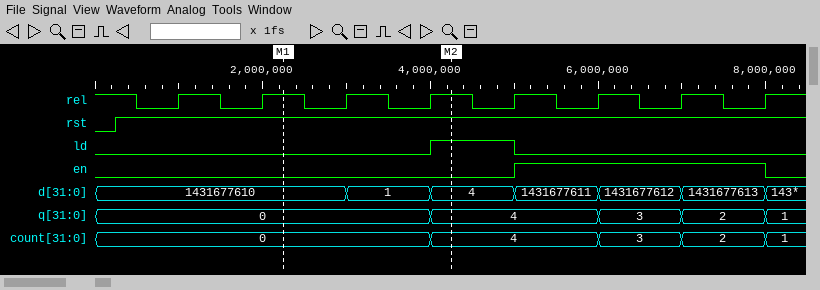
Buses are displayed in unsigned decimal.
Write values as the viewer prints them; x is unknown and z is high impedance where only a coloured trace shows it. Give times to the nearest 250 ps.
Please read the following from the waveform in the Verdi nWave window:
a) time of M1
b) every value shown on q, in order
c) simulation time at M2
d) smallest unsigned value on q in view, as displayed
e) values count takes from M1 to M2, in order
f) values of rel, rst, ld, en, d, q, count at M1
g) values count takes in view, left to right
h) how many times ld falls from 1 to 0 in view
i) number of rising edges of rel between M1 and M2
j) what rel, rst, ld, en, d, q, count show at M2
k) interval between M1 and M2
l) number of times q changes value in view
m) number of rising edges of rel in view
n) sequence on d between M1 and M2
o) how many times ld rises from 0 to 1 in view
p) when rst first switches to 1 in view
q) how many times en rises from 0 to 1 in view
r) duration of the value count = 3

2250 ps
0, 4, 3, 2, 1
4250 ps
0
0, 4
rel=1, rst=1, ld=0, en=0, d=1431677610, q=0, count=0
0, 4, 3, 2, 1
1
2
rel=1, rst=1, ld=1, en=0, d=4, q=4, count=4
2000 ps
4
8
1431677610, 1, 4
1
250 ps
1
1000 ps
